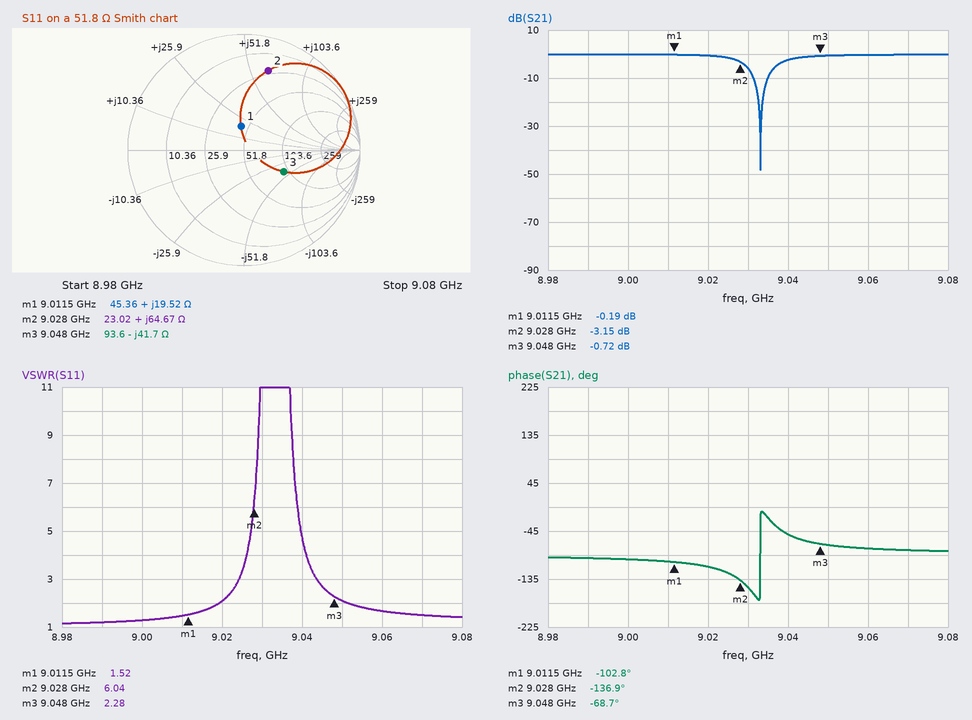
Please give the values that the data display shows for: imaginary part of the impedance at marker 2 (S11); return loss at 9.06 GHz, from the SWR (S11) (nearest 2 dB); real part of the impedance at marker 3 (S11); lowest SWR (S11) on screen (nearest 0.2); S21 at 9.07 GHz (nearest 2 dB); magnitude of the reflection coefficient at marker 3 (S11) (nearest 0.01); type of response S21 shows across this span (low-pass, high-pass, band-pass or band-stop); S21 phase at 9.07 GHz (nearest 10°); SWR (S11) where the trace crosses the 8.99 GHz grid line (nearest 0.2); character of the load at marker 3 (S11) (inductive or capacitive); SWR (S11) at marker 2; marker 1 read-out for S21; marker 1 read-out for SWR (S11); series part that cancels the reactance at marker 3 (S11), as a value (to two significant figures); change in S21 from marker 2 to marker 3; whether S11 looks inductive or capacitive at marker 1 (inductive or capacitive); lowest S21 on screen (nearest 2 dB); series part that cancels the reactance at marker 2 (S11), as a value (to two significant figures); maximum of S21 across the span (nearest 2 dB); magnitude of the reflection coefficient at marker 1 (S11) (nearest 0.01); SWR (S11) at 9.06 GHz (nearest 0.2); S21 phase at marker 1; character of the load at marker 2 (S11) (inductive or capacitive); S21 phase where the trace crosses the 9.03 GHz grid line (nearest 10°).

+64.67 Ω
12 dB
93.6 Ω
1.2
0 dB
0.39
band-stop
-80°
1.2
capacitive
6.04
-0.19 dB
1.52
730 pH
2.43 dB
inductive
-48 dB
270 fF
0 dB
0.21
1.6
-102.8°
inductive
-150°
